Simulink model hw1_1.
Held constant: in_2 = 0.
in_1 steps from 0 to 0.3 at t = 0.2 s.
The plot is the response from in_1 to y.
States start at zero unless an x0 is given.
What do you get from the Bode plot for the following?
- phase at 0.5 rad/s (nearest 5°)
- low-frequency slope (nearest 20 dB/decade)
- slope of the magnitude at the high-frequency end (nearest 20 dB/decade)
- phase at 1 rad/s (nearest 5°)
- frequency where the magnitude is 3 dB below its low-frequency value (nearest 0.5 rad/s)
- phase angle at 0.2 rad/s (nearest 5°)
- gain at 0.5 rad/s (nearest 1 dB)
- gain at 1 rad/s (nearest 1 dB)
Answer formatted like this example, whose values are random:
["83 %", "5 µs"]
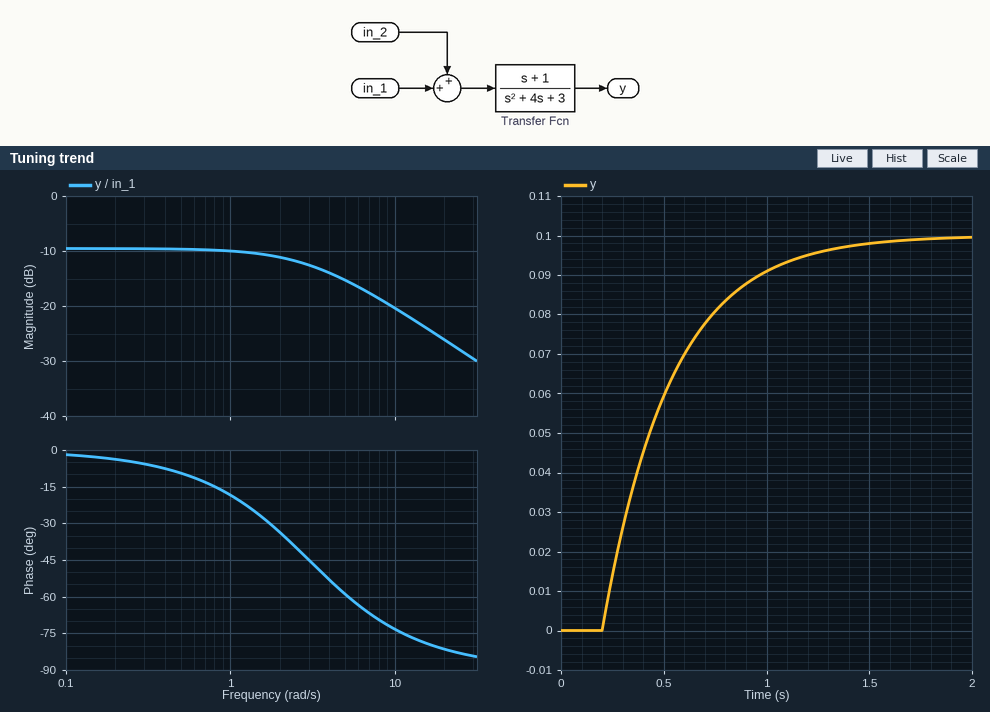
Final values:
["-10°", "0 dB/decade", "-20 dB/decade", "-20°", "3.0 rad/s", "-5°", "-10 dB", "-10 dB"]
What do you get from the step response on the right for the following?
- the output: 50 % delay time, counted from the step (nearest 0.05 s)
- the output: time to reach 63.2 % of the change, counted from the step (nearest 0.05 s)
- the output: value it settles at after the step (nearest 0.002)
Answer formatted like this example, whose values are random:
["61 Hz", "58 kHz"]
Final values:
["0.25 s", "0.35 s", "0.100"]
